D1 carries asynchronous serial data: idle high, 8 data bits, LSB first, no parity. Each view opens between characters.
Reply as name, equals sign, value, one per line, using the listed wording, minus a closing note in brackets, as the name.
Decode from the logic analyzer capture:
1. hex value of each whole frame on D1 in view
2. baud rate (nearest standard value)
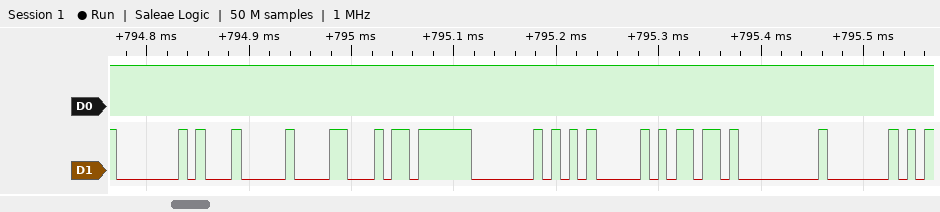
hex value of each whole frame on D1 in view = 40, 04, 18, FB, 40, 05, 6D, 00, 40
baud rate = 115200 baud
